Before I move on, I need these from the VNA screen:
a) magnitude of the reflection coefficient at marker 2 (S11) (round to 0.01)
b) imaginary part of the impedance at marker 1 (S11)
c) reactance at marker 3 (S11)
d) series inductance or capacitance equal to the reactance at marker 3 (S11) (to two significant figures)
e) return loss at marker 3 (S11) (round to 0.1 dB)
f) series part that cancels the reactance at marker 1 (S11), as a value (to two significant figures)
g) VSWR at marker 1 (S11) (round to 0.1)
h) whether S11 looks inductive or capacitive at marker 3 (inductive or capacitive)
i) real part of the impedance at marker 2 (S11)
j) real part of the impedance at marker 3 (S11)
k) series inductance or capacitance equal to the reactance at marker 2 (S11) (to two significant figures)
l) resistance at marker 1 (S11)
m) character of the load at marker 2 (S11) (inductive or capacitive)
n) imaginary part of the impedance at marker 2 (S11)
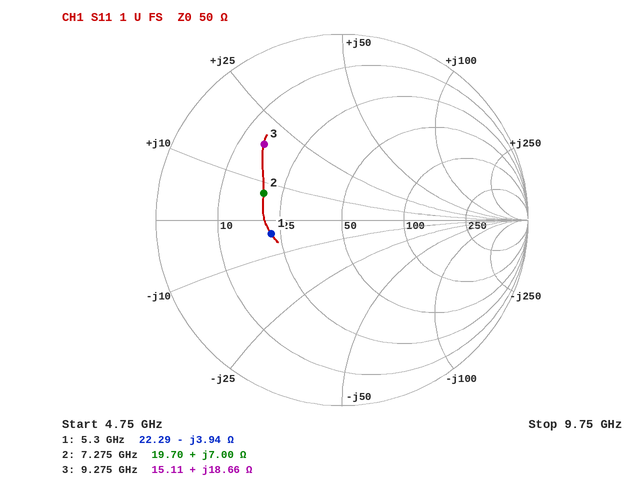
0.44
-3.94 Ω
+18.66 Ω
320 pH
4.7 dB
120 pH
2.3
inductive
19.70 Ω
15.11 Ω
150 pH
22.29 Ω
inductive
+7.00 Ω
